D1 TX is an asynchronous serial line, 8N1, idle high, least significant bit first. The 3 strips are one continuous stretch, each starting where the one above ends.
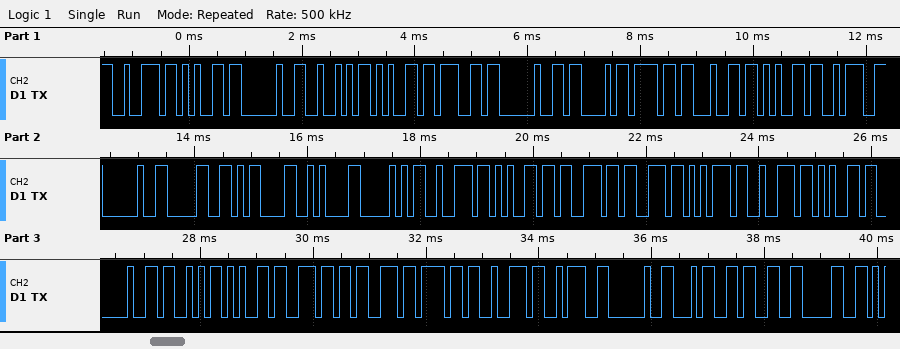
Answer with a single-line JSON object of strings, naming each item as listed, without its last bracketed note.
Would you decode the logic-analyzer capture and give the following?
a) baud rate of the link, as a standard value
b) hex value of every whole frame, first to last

{"baud rate of the link, as a standard value": "9600 baud", "hex value of every whole frame, first to last": "0x72 0x65 0x20 0x52 0x65 0x67 0x20 0x43 0x6F 0x64 0x65 0x3A 0x20 0x30 0x0D 0x0A 0x50 0x72 0x65 0x73 0x73 0x75 0x72 0x65 0x20 0x53 0x65 0x6E 0x73 0x6F 0x72 0x3A 0x20 0x34 0x33 0x30"}
